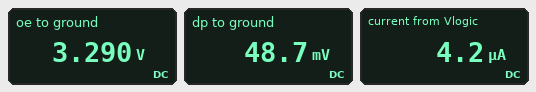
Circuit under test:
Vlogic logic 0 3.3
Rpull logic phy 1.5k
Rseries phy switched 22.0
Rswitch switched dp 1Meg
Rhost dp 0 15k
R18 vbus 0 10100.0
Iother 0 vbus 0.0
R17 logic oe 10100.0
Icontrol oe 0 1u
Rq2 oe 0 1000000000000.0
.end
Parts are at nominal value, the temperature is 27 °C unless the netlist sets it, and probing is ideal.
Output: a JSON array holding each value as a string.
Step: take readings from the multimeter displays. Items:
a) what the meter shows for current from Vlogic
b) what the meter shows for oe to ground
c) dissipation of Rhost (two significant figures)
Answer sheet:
["4.2 µA", "3.290 V", "160 nW"]
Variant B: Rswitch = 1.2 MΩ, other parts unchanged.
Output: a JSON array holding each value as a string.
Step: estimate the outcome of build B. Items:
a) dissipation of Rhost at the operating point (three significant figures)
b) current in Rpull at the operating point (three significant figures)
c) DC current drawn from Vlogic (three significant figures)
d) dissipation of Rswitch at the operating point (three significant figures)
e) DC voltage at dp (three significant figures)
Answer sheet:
["110 nW", "2.71 µA", "3.71 µA", "8.83 µW", "40.7 mV"]
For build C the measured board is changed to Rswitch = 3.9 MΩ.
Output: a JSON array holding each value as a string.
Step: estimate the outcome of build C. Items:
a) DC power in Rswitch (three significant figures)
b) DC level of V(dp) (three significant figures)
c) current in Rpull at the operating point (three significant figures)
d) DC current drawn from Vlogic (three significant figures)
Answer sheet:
["2.77 µW", "12.6 mV", "843 nA", "1.84 µA"]
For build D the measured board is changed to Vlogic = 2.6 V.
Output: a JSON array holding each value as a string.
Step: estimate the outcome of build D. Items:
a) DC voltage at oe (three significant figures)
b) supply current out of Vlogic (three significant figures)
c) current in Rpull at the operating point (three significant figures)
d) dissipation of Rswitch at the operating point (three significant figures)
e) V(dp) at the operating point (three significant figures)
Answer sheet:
["2.59 V", "3.56 µA", "2.56 µA", "6.54 µW", "38.4 mV"]
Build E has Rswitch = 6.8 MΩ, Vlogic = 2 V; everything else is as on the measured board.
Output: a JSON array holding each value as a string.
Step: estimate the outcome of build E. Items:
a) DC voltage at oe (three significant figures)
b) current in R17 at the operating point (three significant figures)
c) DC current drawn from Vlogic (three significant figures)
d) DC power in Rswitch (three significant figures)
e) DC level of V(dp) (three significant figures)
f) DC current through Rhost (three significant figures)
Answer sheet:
["1.99 V", "1.00 µA", "1.29 µA", "585 nW", "4.40 mV", "293 nA"]
